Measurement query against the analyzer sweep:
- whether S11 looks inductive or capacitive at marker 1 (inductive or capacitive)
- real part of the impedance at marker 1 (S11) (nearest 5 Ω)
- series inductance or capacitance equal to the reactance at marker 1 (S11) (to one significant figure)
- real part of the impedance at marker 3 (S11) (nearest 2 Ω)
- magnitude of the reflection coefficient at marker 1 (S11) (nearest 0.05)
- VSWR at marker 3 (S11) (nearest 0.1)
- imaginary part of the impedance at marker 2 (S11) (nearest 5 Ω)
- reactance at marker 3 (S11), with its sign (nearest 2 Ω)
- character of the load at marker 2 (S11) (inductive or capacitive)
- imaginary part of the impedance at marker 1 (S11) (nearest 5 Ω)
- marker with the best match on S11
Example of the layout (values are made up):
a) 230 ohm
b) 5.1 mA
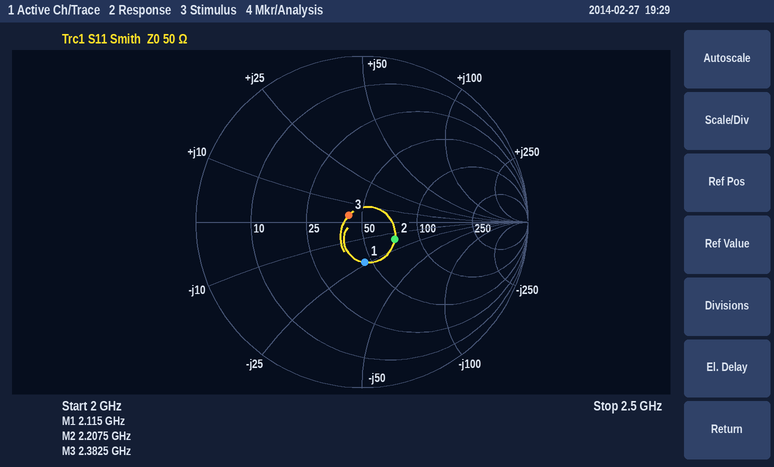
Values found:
a) capacitive
b) 45 Ω
c) 3 pF
d) 42 Ω
e) 0.25
f) 1.2
g) -15 Ω
h) +4 Ω
i) capacitive
j) -25 Ω
k) marker 3
